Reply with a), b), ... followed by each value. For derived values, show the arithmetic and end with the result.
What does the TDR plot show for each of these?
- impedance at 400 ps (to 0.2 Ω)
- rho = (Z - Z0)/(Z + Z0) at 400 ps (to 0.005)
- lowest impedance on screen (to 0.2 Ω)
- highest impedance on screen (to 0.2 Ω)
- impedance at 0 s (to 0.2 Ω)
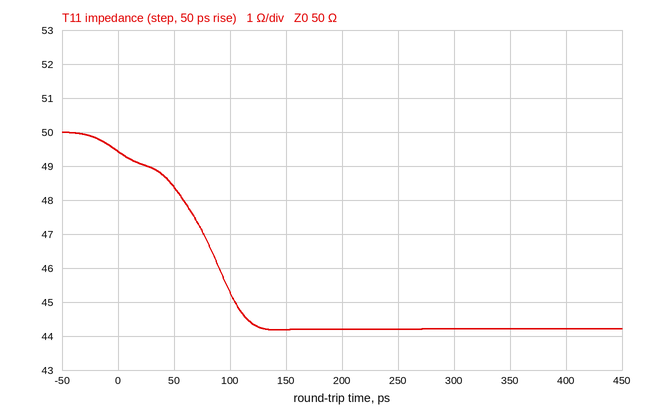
a) 44.2 Ω
b) (44.2 − 50)/(44.2 + 50) ≈ -0.0616, so -0.060 to the nearest 0.005
c) 44.2 Ω
d) 50.0 Ω
e) 49.4 Ω
